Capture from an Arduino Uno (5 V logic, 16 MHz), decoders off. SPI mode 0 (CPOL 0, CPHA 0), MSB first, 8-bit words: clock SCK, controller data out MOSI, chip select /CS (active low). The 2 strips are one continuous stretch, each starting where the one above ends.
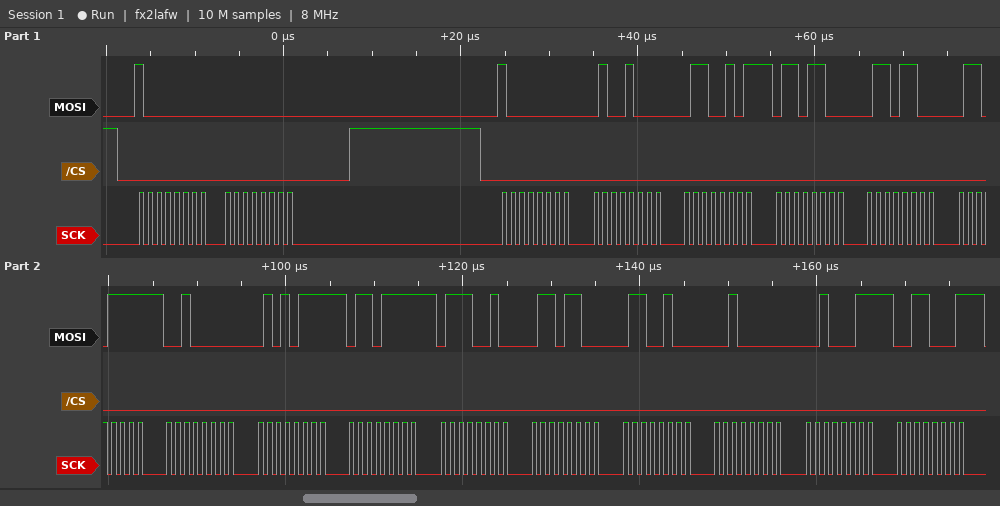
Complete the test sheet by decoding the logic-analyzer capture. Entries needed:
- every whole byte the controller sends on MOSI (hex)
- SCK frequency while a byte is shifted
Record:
80 00 80 48 65 6C 6C 6F 20 57 6F 72 6C 64 20 23 31
1 MHz
